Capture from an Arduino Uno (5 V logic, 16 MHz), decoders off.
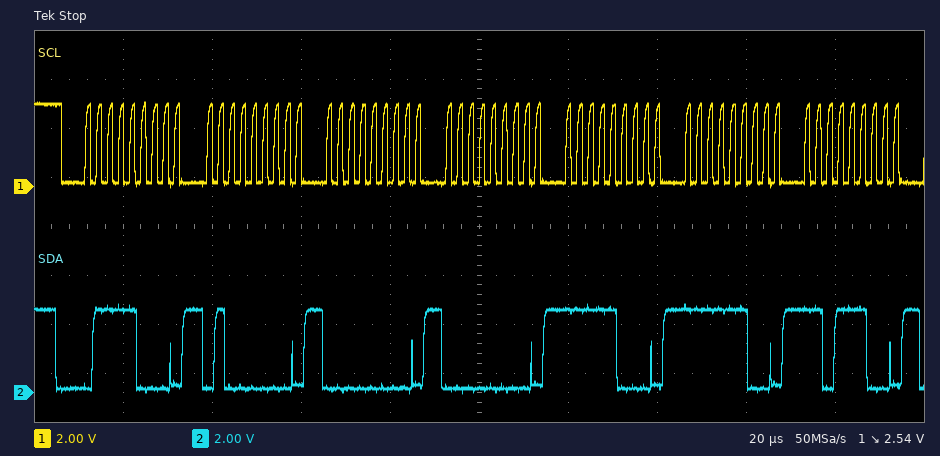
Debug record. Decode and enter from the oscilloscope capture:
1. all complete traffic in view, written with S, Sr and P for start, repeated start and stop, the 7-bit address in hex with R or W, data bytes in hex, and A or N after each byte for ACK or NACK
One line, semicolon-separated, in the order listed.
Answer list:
S 3CW A 40 A 00 A 00 A F8 A FC A DC A
